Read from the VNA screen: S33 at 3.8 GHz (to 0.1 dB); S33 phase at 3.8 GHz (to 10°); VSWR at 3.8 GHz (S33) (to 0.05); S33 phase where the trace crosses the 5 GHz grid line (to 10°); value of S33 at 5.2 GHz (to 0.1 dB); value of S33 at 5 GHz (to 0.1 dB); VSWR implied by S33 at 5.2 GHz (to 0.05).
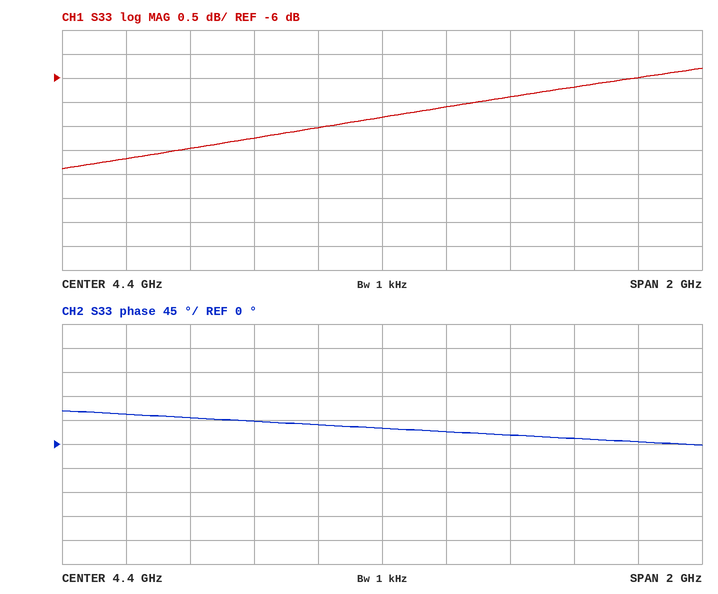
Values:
-7.5 dB
50°
2.45
10°
-6.0 dB
-6.2 dB
3.00
